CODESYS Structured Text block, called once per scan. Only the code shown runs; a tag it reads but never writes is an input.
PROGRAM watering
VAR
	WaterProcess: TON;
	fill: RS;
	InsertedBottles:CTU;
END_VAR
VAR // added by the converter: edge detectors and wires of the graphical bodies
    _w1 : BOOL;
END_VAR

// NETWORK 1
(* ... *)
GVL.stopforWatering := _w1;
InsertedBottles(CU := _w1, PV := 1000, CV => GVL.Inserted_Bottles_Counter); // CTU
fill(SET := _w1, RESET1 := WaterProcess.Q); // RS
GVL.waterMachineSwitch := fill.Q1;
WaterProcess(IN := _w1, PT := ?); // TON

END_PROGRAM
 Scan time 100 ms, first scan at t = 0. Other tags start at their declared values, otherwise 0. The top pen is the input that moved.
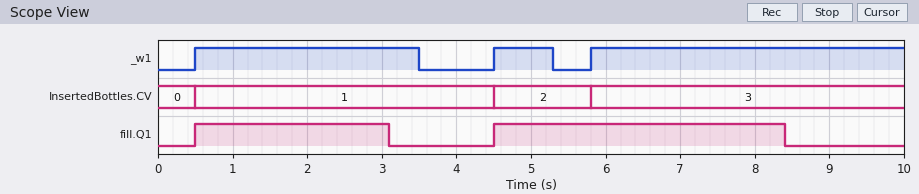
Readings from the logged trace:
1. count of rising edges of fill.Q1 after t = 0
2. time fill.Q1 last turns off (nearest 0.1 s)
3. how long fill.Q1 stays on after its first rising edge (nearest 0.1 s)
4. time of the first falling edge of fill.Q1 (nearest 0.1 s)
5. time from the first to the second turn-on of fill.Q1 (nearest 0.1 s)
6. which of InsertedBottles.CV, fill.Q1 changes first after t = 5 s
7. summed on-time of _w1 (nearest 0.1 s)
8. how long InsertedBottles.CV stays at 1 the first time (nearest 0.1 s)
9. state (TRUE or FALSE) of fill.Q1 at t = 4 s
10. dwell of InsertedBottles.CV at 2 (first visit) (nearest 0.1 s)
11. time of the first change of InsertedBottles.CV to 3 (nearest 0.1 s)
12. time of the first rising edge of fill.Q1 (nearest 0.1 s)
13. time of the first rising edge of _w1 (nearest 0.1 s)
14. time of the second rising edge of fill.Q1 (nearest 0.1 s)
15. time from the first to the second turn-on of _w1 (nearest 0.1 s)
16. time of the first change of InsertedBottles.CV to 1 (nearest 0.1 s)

2
8.4 s
2.6 s
3.1 s
4.0 s
InsertedBottles.CV
8.0 s
4.0 s
FALSE
1.3 s
5.8 s
0.5 s
0.5 s
4.5 s
4.0 s
0.5 s
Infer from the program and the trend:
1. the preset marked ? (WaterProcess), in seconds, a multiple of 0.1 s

2.5 s
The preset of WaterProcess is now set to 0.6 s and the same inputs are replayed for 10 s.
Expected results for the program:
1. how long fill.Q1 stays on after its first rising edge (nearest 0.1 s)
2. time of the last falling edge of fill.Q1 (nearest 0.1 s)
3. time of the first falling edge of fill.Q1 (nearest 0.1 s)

0.7 s
6.5 s
1.2 s
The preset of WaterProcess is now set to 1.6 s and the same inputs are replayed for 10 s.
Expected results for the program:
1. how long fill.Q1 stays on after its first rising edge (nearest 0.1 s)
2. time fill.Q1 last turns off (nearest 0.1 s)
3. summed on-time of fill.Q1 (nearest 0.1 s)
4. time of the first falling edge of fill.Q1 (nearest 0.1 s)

1.7 s
7.5 s
4.7 s
2.2 s
